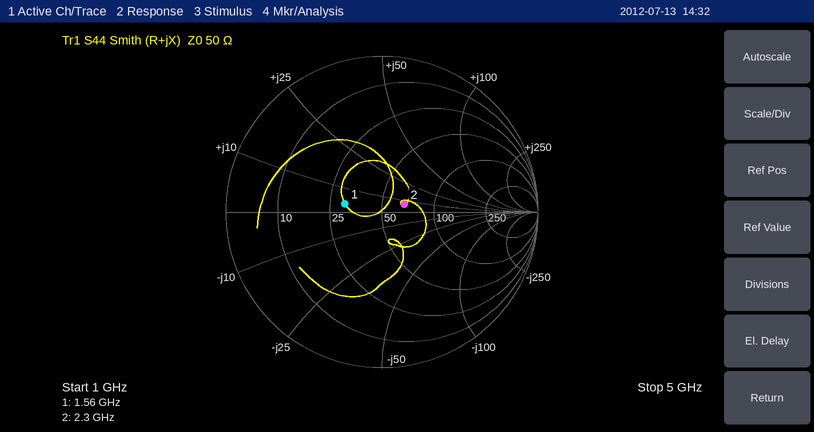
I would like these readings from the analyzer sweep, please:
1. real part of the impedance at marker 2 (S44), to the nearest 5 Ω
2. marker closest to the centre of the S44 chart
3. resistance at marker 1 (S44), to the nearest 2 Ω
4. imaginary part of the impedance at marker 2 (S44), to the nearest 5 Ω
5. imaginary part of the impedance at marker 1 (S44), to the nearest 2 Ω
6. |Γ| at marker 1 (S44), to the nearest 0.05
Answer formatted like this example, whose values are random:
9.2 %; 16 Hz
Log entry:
65 Ω; marker 2; 30 Ω; +5 Ω; +4 Ω; 0.25
